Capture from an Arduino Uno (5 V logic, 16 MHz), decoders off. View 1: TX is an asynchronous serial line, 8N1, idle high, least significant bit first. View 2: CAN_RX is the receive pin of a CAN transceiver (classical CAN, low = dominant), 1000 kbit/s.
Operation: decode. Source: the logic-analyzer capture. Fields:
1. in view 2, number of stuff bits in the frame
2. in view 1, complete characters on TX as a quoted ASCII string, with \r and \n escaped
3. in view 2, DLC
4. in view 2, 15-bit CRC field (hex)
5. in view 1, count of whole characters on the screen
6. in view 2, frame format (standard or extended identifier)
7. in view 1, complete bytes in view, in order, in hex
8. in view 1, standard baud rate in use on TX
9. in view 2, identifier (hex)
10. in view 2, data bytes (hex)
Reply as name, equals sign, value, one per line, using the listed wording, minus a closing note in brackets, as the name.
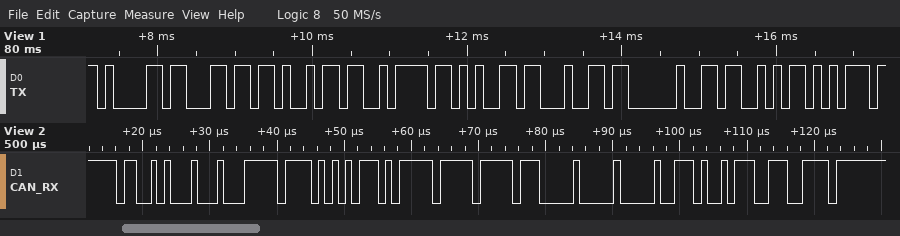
in view 2, number of stuff bits in the frame = 7
in view 1, complete characters on TX as a quoted ASCII string, with \r and \n escaped = "alized Su"
in view 2, DLC = 8
in view 2, 15-bit CRC field = 0x5CE7
in view 1, count of whole characters on the screen = 9
in view 2, frame format = standard
in view 1, complete bytes in view, in order, in hex = 0x61 0x6C 0x69 0x7A 0x65 0x64 0x20 0x53 0x75
in view 1, standard baud rate in use on TX = 9600 baud
in view 2, identifier = 0x651
in view 2, data bytes = FF AA EB FF FF 00 00 74
